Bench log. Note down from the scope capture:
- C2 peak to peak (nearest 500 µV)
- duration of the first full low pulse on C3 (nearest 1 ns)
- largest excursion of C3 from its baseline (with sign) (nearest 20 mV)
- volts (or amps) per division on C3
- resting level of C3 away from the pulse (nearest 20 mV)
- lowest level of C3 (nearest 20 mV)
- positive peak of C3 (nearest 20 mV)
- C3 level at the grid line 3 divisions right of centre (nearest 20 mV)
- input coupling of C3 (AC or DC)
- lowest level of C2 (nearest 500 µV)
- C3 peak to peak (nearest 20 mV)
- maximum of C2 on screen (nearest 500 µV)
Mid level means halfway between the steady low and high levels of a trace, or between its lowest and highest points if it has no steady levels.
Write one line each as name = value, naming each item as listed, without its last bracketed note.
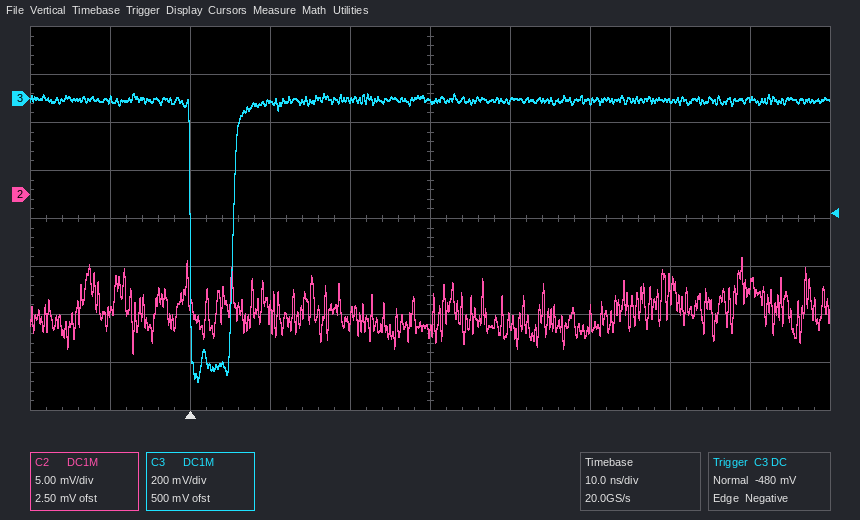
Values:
C2 peak to peak = 10.0 mV
duration of the first full low pulse on C3 = 5 ns
largest excursion of C3 from its baseline (with sign) = -1.18 V
volts (or amps) per division on C3 = 200 mV
resting level of C3 away from the pulse = 0 mV
lowest level of C3 = -1.18 V
positive peak of C3 = 20 mV
C3 level at the grid line 3 divisions right of centre = 0 mV
input coupling of C3 = DC
lowest level of C2 = -16.5 mV
C3 peak to peak = 1.20 V
maximum of C2 on screen = -6.5 mV
